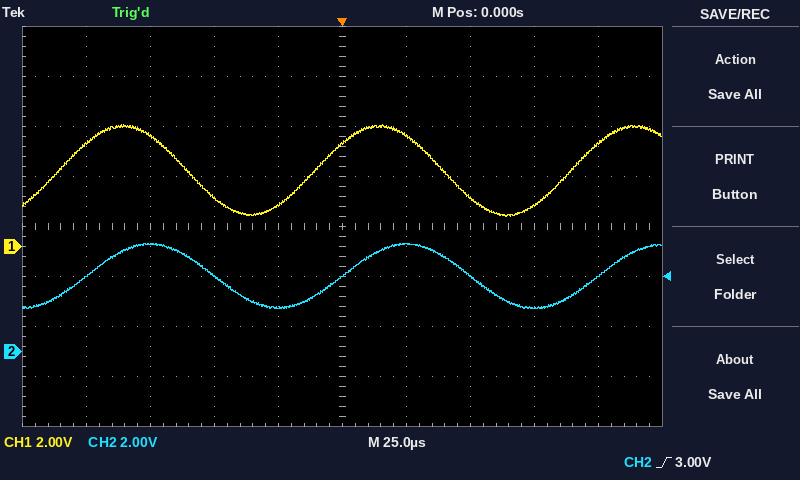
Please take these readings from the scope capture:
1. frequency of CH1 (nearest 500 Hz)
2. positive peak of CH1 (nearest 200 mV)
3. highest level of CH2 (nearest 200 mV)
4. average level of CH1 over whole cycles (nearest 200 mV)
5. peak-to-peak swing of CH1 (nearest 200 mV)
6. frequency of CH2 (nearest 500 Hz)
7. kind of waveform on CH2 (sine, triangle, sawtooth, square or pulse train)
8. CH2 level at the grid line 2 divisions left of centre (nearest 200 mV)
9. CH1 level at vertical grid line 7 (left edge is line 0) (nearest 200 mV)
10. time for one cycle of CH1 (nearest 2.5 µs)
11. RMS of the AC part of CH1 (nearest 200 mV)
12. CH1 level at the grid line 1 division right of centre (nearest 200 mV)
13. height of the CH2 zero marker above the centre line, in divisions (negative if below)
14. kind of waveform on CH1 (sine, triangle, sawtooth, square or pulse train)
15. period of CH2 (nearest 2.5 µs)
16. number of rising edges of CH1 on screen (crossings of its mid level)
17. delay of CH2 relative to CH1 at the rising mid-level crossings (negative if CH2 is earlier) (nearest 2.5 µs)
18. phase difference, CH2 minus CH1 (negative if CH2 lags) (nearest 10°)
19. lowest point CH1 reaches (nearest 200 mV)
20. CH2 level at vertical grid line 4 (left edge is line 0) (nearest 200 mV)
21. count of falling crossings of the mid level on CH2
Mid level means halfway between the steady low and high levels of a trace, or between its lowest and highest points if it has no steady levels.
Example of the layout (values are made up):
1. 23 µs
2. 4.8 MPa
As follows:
1. 10.0 kHz
2. 4.8 V
3. 4.4 V
4. 3.0 V
5. 3.6 V
6. 10.0 kHz
7. sine
8. 3.0 V
9. 2.0 V
10. 100.0 µs
11. 1.2 V
12. 4.4 V
13. -2.5 div
14. sine
15. 100.0 µs
16. 3
17. +10.0 µs
18. -40°
19. 1.2 V
20. 1.8 V
21. 2
